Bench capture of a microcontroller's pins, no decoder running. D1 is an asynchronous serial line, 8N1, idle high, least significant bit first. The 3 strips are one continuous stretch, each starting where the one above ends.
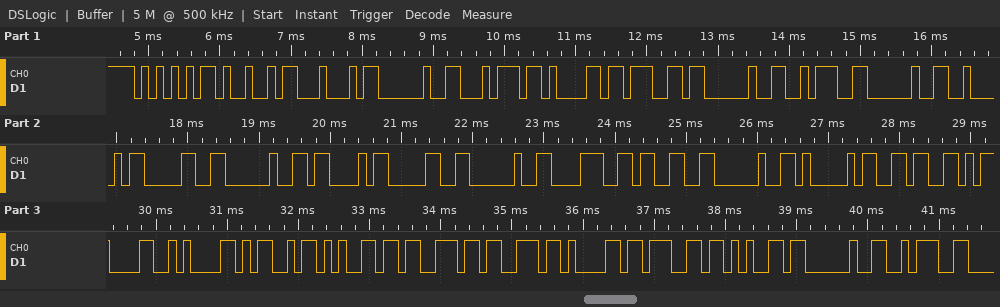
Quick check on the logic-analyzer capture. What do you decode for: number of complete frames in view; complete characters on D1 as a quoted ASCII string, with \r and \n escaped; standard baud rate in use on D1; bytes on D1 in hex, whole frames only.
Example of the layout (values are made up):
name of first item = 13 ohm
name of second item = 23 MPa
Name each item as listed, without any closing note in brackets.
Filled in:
number of complete frames in view = 32
complete characters on D1 as a quoted ASCII string, with \r and \n escaped = "UID tag : B0 C0 83 A6\r\nMessage :"
standard baud rate in use on D1 = 9600 baud
bytes on D1 in hex, whole frames only = 55 49 44 20 74 61 67 20 3A 20 42 30 20 43 30 20 38 33 20 41 36 0D 0A 4D 65 73 73 61 67 65 20 3A
